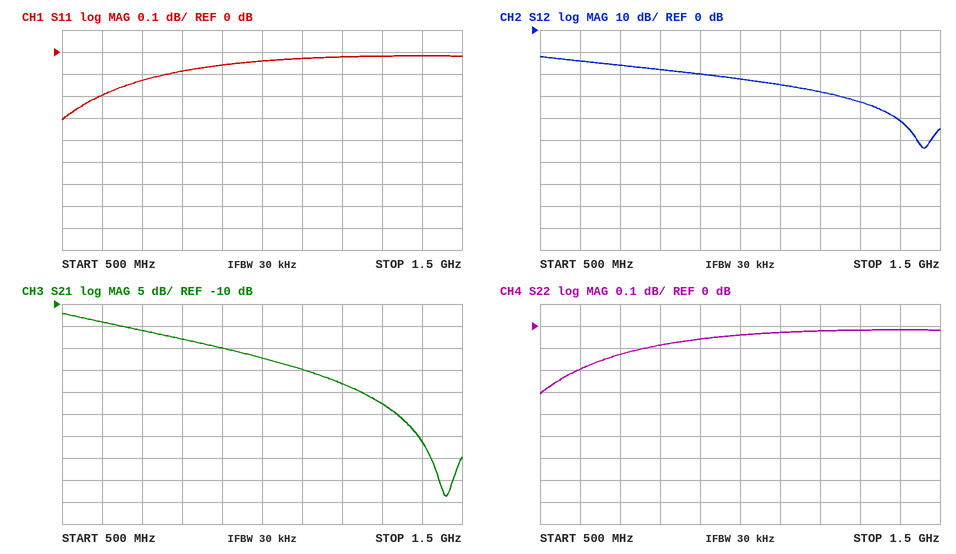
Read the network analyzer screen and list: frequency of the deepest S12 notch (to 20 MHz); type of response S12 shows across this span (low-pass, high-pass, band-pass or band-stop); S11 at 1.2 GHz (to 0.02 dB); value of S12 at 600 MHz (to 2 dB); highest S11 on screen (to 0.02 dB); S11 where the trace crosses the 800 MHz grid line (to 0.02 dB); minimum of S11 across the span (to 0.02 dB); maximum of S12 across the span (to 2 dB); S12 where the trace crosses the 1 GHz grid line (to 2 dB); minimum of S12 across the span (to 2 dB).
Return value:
1.46 GHz
low-pass
-0.02 dB
-14 dB
-0.02 dB
-0.08 dB
-0.30 dB
-12 dB
-22 dB
-54 dB
